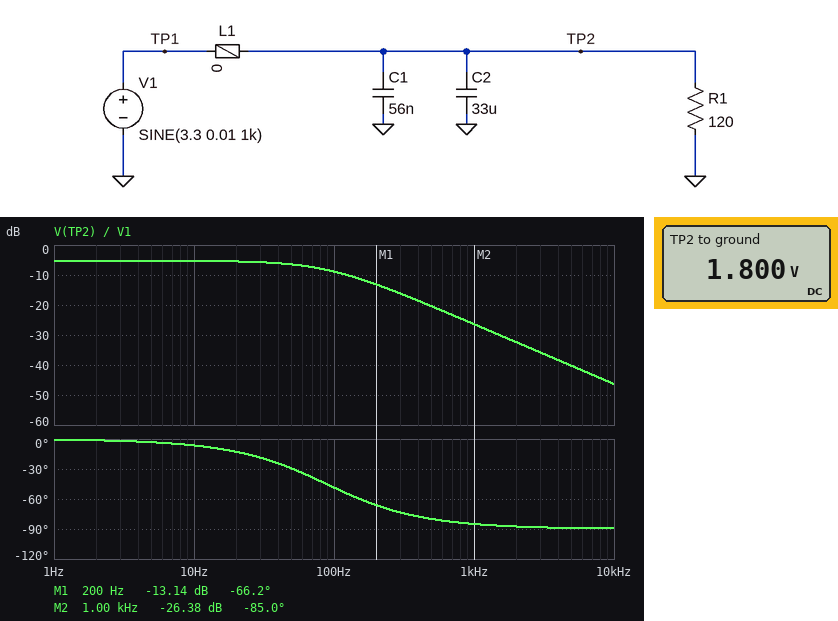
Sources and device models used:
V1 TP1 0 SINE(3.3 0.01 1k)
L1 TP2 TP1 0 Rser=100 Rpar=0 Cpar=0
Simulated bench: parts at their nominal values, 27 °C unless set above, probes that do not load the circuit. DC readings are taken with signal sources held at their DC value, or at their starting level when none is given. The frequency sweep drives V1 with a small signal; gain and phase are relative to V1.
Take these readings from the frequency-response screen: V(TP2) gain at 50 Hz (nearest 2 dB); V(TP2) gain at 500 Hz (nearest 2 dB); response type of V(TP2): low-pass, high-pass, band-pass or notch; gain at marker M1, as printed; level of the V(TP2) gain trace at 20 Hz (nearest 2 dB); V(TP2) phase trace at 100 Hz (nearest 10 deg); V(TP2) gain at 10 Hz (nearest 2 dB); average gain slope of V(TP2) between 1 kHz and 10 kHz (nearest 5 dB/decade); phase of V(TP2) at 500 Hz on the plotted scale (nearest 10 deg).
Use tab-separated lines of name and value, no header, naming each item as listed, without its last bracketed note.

V(TP2) gain at 50 Hz	-6 dB
V(TP2) gain at 500 Hz	-20 dB
response type of V(TP2): low-pass, high-pass, band-pass or notch	low-pass
gain at marker M1, as printed	-13.14 dB
level of the V(TP2) gain trace at 20 Hz	-6 dB
V(TP2) phase trace at 100 Hz	-50 deg
V(TP2) gain at 10 Hz	-6 dB
average gain slope of V(TP2) between 1 kHz and 10 kHz	-20 dB/decade
phase of V(TP2) at 500 Hz on the plotted scale	-80 deg
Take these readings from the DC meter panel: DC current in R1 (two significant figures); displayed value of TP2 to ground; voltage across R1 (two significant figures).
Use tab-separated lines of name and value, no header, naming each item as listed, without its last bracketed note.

DC current in R1	15 mA
displayed value of TP2 to ground	1.800 V
voltage across R1	1.8 V
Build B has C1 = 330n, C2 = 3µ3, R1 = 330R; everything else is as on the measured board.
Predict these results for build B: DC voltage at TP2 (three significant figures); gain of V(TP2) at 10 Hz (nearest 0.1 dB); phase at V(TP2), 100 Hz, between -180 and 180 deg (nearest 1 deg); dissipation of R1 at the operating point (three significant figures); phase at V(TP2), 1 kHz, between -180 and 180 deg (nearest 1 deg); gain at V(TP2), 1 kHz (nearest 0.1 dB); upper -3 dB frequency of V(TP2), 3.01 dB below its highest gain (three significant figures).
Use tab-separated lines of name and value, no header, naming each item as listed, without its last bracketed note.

DC voltage at TP2	2.53 V
gain of V(TP2) at 10 Hz	-2.3 dB
phase at V(TP2), 100 Hz, between -180 and 180 deg	-10 deg
dissipation of R1 at the operating point	19.4 mW
phase at V(TP2), 1 kHz, between -180 and 180 deg	-60 deg
gain at V(TP2), 1 kHz	-8.4 dB
upper -3 dB frequency of V(TP2), 3.01 dB below its highest gain	571 Hz
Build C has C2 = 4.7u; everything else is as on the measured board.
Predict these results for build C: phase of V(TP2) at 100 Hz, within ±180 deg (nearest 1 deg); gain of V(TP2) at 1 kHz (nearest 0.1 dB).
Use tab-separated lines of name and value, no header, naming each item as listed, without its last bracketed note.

phase of V(TP2) at 100 Hz, within ±180 deg	-9 deg
gain of V(TP2) at 1 kHz	-10.9 dB
